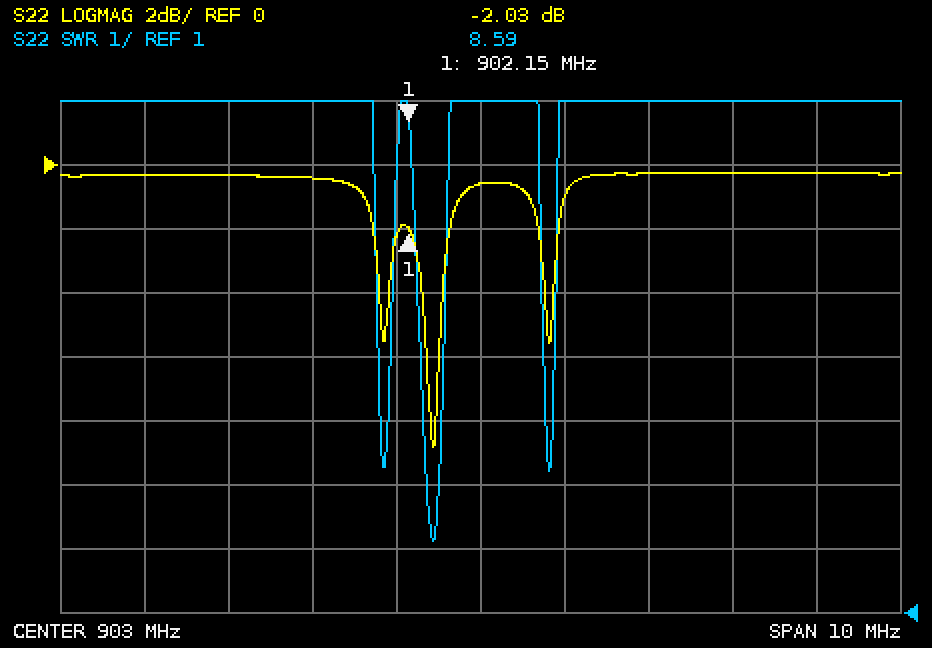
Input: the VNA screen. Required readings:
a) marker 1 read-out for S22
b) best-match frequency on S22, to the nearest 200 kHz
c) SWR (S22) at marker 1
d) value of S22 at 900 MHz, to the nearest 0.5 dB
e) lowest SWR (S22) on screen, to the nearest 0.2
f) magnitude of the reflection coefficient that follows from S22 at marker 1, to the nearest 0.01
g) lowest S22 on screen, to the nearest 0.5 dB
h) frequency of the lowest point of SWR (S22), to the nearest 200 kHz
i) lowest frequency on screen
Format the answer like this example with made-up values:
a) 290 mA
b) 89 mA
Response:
a) -2.03 dB
b) 902.4 MHz
c) 8.59
d) -0.5 dB
e) 2.2
f) 0.79
g) -9.0 dB
h) 902.4 MHz
i) 898 MHz
